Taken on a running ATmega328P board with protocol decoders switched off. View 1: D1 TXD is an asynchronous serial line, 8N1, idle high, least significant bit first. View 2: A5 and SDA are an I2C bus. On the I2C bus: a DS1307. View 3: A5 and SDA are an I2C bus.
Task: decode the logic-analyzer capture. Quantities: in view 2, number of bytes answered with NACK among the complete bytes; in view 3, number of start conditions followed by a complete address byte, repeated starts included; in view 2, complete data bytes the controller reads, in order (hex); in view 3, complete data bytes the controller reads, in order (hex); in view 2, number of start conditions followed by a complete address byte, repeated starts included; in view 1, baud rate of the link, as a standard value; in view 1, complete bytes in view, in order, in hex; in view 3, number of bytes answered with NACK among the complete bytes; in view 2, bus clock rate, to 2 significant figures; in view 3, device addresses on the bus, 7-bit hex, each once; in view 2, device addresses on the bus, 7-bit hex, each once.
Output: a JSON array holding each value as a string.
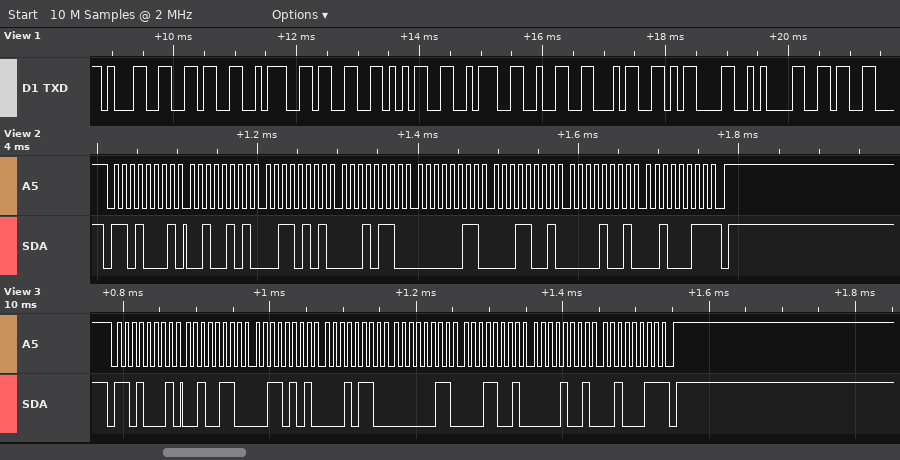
["1", "1", "25 35 16 03 19 09 23", "26 35 16 03 19 09 23", "1", "9600 baud", "31 36 3A 33 35 3A 32 34 0D 0A 36", "1", "100 kHz", "0x68", "0x68"]
